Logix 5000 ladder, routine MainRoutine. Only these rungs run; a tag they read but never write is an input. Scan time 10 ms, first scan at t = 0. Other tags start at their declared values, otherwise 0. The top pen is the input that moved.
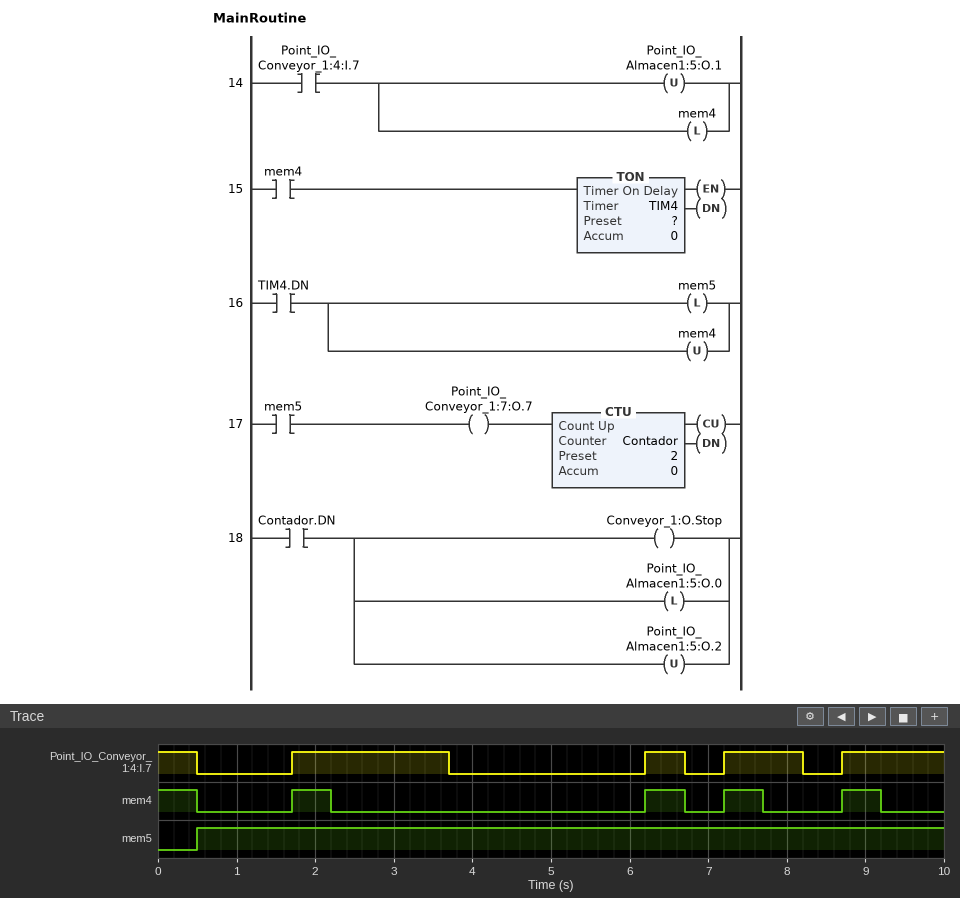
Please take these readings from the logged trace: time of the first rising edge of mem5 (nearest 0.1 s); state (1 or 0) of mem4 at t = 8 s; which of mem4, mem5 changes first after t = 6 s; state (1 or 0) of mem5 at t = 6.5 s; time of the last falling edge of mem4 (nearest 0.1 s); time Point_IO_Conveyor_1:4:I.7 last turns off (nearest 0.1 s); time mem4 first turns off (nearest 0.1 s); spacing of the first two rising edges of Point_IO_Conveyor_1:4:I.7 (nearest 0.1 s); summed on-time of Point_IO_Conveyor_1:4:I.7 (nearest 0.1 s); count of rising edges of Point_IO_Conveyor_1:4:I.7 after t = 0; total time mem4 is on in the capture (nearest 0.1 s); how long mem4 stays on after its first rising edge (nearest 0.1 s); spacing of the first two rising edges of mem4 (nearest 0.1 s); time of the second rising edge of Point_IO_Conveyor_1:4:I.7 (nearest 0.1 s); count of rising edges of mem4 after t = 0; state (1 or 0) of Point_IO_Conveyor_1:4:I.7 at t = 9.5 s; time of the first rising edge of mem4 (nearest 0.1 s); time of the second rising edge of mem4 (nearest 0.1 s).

0.5 s
0
mem4
1
9.2 s
8.2 s
0.5 s
4.5 s
5.3 s
4
2.5 s
0.5 s
4.5 s
6.2 s
4
1
1.7 s
6.2 s
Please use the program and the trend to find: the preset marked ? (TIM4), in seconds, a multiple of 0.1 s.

0.5 s
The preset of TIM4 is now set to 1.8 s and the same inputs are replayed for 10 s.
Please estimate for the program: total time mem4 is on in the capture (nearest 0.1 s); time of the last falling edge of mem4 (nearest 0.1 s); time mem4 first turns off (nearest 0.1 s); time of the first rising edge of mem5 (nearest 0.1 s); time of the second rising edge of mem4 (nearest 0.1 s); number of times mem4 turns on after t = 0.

4.9 s
8.0 s
1.8 s
1.8 s
8.7 s
2
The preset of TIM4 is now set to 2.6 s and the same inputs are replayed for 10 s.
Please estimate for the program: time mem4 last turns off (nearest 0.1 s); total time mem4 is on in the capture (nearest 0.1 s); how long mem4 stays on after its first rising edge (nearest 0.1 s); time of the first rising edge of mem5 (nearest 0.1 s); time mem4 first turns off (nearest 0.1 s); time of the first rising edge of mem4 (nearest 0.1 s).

8.8 s
5.2 s
2.6 s
2.6 s
2.6 s
6.2 s
